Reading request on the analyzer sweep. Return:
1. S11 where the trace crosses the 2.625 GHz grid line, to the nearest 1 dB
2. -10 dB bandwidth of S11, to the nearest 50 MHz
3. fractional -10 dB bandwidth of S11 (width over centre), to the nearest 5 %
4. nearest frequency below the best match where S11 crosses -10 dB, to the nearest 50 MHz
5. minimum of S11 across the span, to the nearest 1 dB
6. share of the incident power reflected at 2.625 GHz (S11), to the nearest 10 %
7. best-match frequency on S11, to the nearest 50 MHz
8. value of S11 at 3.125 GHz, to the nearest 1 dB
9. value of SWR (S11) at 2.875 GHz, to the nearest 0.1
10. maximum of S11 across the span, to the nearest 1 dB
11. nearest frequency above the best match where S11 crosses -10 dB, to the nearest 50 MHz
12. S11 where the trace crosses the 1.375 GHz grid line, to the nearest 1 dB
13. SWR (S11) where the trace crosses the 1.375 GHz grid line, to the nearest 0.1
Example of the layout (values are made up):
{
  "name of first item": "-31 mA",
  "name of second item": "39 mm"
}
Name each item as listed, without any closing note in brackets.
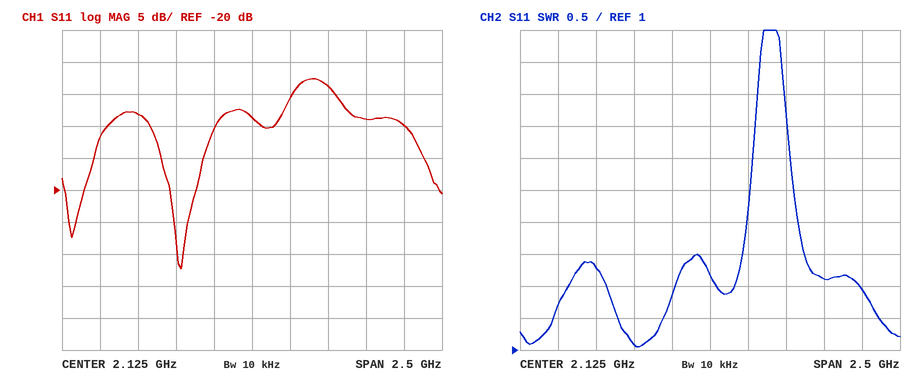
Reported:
{
  "S11 where the trace crosses the 2.625 GHz grid line, to the nearest 1 dB": "-4 dB",
  "-10 dB bandwidth of S11, to the nearest 50 MHz": "450 MHz",
  "fractional -10 dB bandwidth of S11 (width over centre), to the nearest 5 %": "25 %",
  "nearest frequency below the best match where S11 crosses -10 dB, to the nearest 50 MHz": "1.45 GHz",
  "minimum of S11 across the span, to the nearest 1 dB": "-32 dB",
  "share of the incident power reflected at 2.625 GHz (S11), to the nearest 10 %": "40 %",
  "best-match frequency on S11, to the nearest 50 MHz": "1.65 GHz",
  "value of S11 at 3.125 GHz, to the nearest 1 dB": "-10 dB",
  "value of SWR (S11) at 2.875 GHz, to the nearest 0.1": "2.1",
  "maximum of S11 across the span, to the nearest 1 dB": "-3 dB",
  "nearest frequency above the best match where S11 crosses -10 dB, to the nearest 50 MHz": "1.90 GHz",
  "S11 where the trace crosses the 1.375 GHz grid line, to the nearest 1 dB": "-8 dB",
  "SWR (S11) where the trace crosses the 1.375 GHz grid line, to the nearest 0.1": "2.3"
}
